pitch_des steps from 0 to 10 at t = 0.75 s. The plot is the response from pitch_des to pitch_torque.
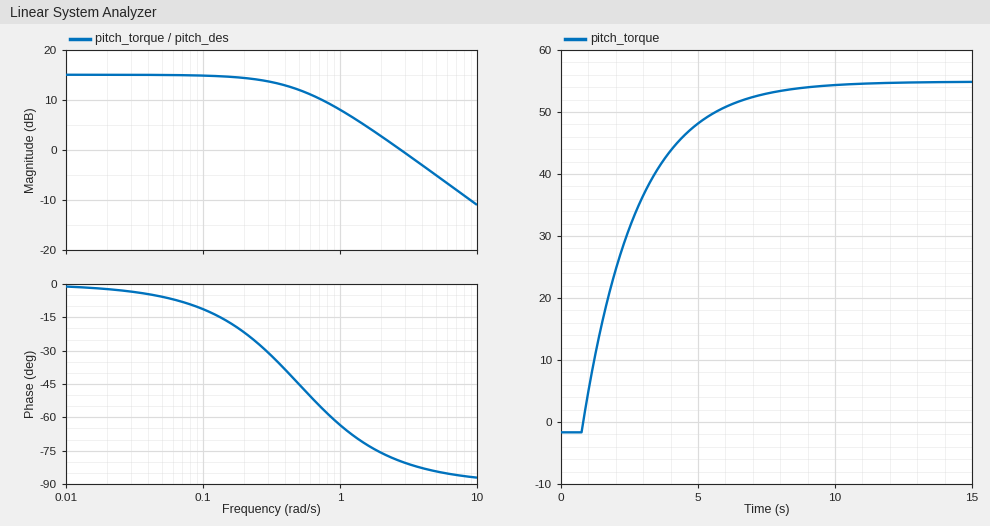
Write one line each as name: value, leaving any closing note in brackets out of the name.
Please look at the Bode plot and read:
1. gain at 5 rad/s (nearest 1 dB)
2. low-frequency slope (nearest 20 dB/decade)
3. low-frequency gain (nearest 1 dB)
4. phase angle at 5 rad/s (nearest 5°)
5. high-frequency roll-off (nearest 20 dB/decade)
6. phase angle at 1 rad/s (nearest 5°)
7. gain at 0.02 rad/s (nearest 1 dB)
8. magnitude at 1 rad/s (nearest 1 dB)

gain at 5 rad/s: -5 dB
low-frequency slope: 0 dB/decade
low-frequency gain: 15 dB
phase angle at 5 rad/s: -85°
high-frequency roll-off: -20 dB/decade
phase angle at 1 rad/s: -65°
gain at 0.02 rad/s: 15 dB
magnitude at 1 rad/s: 8 dB
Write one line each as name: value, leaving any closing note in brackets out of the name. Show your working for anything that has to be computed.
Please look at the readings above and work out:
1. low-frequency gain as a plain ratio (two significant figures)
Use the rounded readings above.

low-frequency gain as a plain ratio: 10^(15 / 20) = 5.6
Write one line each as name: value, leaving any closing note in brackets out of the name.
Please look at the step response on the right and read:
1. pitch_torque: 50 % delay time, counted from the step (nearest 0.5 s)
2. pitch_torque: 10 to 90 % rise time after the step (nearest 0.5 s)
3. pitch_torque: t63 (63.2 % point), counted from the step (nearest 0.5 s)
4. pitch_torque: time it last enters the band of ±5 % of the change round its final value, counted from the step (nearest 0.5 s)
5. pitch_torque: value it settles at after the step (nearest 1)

pitch_torque: 50 % delay time, counted from the step: 1.5 s
pitch_torque: 10 to 90 % rise time after the step: 4.5 s
pitch_torque: t63 (63.2 % point), counted from the step: 2.0 s
pitch_torque: time it last enters the band of ±5 % of the change round its final value, counted from the step: 6.0 s
pitch_torque: value it settles at after the step: 55
